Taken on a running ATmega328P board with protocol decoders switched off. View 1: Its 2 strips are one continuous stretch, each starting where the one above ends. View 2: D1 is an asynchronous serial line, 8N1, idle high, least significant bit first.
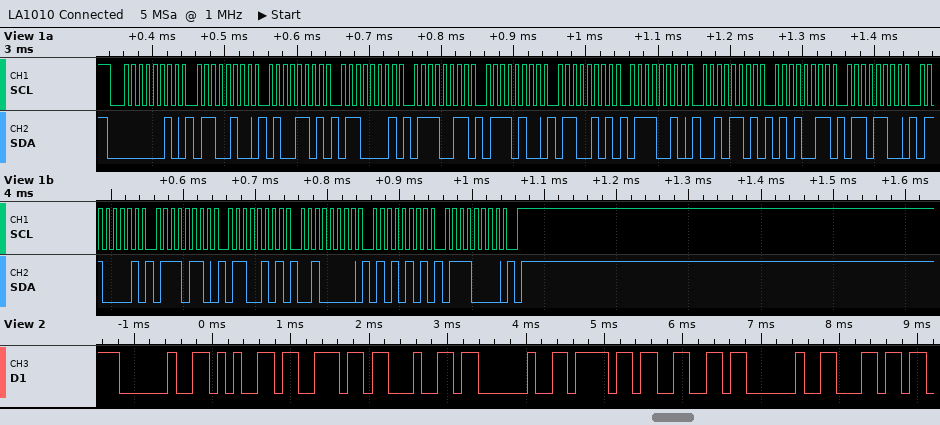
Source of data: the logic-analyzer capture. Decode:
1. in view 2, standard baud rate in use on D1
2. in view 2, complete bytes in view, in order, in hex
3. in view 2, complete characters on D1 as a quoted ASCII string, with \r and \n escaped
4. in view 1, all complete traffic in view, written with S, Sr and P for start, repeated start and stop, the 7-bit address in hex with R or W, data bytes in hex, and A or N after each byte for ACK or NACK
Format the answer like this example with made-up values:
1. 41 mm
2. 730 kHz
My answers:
1. 9600 baud
2. 20 65 6E 64 20 6F 66 20 6C
3. " end of l"
4. S 01W A 64 A 4D A 61 A 73 A 74 A 65 A 72 A 2D A 53 A 6C A 61 A 76 A 65 A 20 A 55 A 70 A P
